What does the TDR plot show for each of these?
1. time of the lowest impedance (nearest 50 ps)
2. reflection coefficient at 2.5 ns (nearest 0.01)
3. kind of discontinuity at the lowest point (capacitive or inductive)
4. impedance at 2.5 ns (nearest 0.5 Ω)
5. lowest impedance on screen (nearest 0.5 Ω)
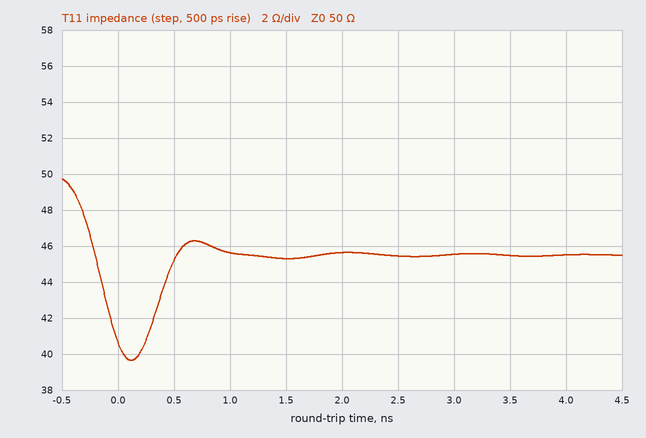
100 ps
-0.05
capacitive
45.5 Ω
39.5 Ω
